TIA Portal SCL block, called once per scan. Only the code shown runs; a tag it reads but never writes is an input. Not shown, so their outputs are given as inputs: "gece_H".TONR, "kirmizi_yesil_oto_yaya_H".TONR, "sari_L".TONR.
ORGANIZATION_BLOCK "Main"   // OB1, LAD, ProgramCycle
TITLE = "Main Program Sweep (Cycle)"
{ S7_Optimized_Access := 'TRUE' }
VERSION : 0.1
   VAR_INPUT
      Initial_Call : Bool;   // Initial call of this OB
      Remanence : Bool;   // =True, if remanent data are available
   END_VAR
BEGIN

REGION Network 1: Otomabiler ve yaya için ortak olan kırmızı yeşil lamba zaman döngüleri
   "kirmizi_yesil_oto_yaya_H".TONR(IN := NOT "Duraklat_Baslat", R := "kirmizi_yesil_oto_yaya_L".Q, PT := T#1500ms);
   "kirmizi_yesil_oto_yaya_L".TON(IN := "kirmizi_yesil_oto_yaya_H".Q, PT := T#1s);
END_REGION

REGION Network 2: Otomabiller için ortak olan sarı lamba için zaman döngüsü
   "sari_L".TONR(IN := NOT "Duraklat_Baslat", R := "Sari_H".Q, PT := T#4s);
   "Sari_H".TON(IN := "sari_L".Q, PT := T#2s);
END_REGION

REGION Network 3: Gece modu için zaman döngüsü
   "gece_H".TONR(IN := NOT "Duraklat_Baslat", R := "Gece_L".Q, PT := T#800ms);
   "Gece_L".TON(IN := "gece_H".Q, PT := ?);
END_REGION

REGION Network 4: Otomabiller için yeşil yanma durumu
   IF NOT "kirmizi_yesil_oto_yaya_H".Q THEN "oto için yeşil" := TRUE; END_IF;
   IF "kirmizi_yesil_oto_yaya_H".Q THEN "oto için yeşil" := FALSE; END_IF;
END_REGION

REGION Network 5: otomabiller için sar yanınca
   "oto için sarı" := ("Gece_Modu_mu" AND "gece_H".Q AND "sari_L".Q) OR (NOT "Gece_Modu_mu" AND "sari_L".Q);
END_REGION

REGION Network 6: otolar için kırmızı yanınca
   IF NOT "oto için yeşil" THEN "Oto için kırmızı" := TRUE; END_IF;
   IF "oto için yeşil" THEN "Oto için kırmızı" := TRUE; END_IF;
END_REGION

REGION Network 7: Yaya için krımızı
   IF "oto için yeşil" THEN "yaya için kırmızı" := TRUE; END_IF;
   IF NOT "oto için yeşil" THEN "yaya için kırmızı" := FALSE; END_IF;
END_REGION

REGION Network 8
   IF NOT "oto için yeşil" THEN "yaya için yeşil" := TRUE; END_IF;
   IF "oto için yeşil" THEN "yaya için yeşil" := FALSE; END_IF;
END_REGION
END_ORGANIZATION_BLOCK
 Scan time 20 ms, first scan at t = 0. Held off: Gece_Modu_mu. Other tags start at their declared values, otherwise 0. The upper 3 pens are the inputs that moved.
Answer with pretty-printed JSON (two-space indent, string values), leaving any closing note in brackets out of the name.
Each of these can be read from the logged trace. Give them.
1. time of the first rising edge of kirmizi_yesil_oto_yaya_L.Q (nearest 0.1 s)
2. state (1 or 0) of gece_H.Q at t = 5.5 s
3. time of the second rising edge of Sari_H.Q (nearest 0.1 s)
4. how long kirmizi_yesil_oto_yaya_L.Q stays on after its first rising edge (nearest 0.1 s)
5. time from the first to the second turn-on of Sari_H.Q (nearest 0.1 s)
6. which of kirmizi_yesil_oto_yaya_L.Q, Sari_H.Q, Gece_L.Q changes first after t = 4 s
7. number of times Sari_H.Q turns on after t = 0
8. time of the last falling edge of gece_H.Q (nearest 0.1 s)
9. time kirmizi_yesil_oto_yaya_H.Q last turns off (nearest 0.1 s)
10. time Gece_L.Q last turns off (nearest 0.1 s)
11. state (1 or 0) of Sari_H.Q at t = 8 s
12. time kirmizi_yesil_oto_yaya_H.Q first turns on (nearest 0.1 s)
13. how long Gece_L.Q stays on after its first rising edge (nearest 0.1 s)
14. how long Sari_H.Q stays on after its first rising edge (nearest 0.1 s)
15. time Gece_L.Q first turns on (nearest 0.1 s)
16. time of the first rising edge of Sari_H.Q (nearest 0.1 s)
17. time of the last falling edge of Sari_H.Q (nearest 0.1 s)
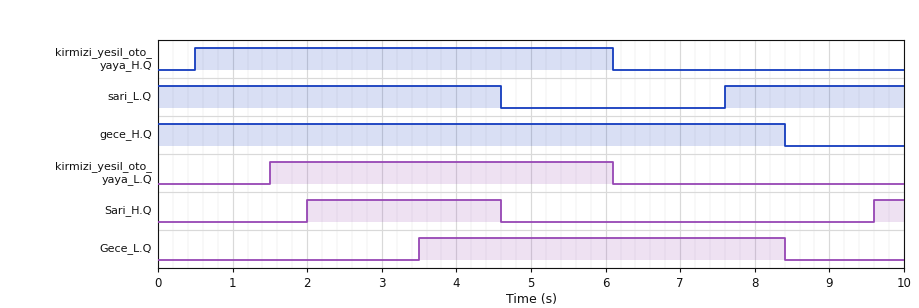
{
  "time of the first rising edge of kirmizi_yesil_oto_yaya_L.Q": "1.5 s",
  "state (1 or 0) of gece_H.Q at t = 5.5 s": "1",
  "time of the second rising edge of Sari_H.Q": "9.6 s",
  "how long kirmizi_yesil_oto_yaya_L.Q stays on after its first rising edge": "4.6 s",
  "time from the first to the second turn-on of Sari_H.Q": "7.6 s",
  "which of kirmizi_yesil_oto_yaya_L.Q, Sari_H.Q, Gece_L.Q changes first after t = 4 s": "Sari_H.Q",
  "number of times Sari_H.Q turns on after t = 0": "2",
  "time of the last falling edge of gece_H.Q": "8.4 s",
  "time kirmizi_yesil_oto_yaya_H.Q last turns off": "6.1 s",
  "time Gece_L.Q last turns off": "8.4 s",
  "state (1 or 0) of Sari_H.Q at t = 8 s": "0",
  "time kirmizi_yesil_oto_yaya_H.Q first turns on": "0.5 s",
  "how long Gece_L.Q stays on after its first rising edge": "4.9 s",
  "how long Sari_H.Q stays on after its first rising edge": "2.6 s",
  "time Gece_L.Q first turns on": "3.5 s",
  "time of the first rising edge of Sari_H.Q": "2.0 s",
  "time of the last falling edge of Sari_H.Q": "4.6 s"
}
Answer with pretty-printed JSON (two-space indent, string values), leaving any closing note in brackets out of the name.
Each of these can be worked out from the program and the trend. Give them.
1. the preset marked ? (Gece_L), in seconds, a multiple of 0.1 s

{
  "the preset marked ? (Gece_L), in seconds, a multiple of 0.1 s": "3.5 s"
}
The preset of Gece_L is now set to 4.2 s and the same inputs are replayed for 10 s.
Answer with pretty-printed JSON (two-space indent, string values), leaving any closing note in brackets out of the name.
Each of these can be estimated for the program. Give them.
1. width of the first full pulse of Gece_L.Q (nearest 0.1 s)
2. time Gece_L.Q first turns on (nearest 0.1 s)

{
  "width of the first full pulse of Gece_L.Q": "4.2 s",
  "time Gece_L.Q first turns on": "4.2 s"
}
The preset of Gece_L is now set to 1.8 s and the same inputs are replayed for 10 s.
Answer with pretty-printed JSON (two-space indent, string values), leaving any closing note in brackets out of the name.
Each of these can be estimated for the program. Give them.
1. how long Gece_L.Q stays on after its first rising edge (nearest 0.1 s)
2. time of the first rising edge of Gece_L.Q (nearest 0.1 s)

{
  "how long Gece_L.Q stays on after its first rising edge": "6.6 s",
  "time of the first rising edge of Gece_L.Q": "1.8 s"
}
